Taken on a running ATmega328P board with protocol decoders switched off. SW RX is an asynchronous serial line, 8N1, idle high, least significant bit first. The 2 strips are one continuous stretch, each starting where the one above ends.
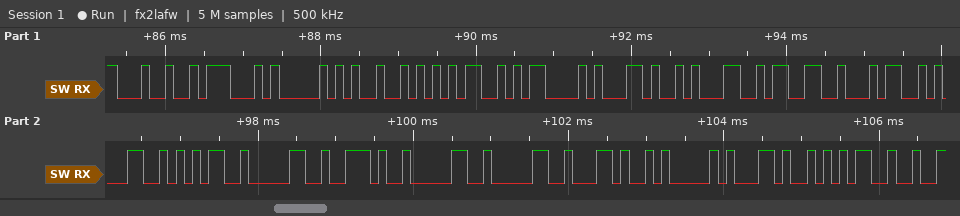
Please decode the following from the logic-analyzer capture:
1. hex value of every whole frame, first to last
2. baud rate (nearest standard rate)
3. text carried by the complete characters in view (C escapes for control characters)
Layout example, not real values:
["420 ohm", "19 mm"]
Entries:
["24 47 50 52 4D 43 2C 31 33 34 31 35 30 2E 30 30 2C 41 2C 35", "9600 baud", "\"$GPRMC,134150.00,A,5\""]
